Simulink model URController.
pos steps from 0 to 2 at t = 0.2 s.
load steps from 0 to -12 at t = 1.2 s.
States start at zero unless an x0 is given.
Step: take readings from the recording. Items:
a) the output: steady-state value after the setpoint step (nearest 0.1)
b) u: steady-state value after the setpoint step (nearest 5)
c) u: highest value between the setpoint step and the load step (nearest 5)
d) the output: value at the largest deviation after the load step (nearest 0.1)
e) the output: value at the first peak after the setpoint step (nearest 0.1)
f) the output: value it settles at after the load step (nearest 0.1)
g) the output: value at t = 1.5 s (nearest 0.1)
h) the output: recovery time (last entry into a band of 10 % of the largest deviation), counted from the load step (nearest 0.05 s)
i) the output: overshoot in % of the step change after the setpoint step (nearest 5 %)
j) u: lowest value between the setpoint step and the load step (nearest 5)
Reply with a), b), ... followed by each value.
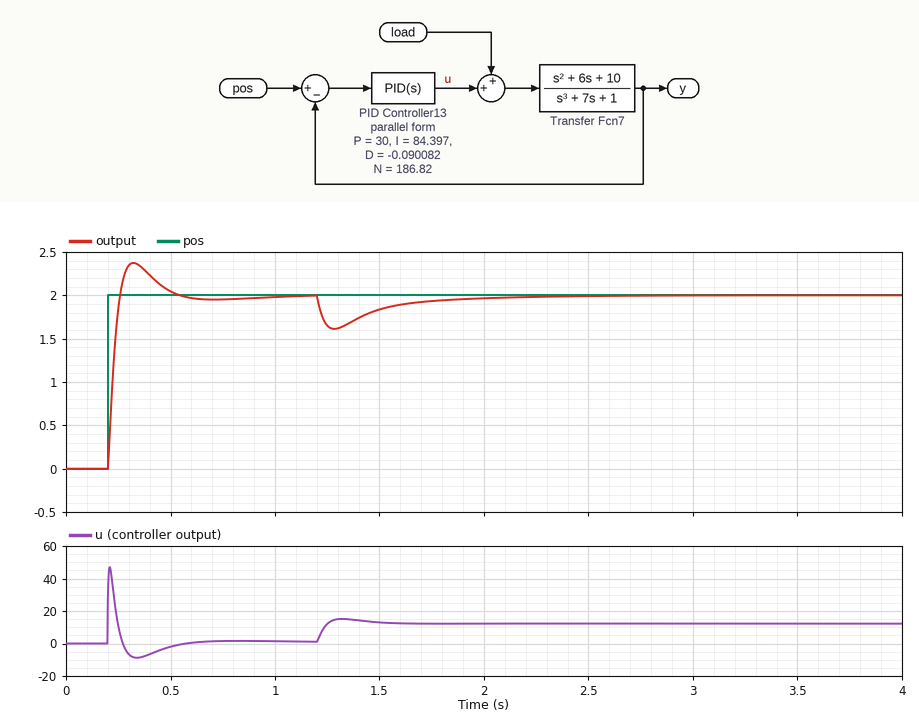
a) 2.0
b) 0
c) 45
d) 1.6
e) 2.4
f) 2.0
g) 1.8
h) 0.75 s
i) 20 %
j) -10
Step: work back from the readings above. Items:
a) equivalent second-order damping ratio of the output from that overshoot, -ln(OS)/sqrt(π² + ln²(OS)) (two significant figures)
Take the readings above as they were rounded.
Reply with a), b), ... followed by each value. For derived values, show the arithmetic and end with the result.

a) ln(0.2) = -1.609; 1.609 / sqrt(9.870 + 2.590) = 0.46
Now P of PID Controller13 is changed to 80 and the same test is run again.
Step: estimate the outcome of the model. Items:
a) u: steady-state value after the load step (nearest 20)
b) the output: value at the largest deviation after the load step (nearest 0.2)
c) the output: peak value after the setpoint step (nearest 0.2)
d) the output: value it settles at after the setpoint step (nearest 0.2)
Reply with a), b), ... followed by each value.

a) 20
b) 1.8
c) 2.2
d) 2.0
